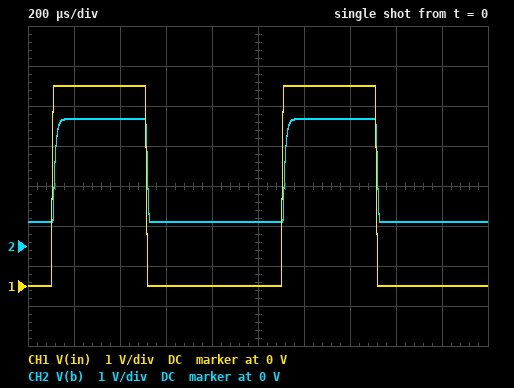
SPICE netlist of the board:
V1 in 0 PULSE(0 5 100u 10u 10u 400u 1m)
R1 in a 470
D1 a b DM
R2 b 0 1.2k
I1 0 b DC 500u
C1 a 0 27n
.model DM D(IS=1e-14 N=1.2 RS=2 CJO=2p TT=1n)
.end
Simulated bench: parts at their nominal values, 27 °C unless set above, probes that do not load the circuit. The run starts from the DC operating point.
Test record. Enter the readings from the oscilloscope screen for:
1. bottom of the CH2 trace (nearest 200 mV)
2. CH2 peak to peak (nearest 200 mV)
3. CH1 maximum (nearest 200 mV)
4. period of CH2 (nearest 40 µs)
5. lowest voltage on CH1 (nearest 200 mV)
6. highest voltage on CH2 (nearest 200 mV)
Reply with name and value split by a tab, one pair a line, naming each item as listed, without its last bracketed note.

bottom of the CH2 trace	600 mV
CH2 peak to peak	2.6 V
CH1 maximum	5.0 V
period of CH2	1.00 ms
lowest voltage on CH1	0 V
highest voltage on CH2	3.2 V
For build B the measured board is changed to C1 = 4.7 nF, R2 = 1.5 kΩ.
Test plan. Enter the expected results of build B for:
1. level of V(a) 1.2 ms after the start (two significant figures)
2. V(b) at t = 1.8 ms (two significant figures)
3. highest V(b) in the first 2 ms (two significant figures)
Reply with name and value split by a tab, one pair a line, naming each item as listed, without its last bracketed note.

level of V(a) 1.2 ms after the start	4.2 V
V(b) at t = 1.8 ms	750 mV
highest V(b) in the first 2 ms	3.4 V
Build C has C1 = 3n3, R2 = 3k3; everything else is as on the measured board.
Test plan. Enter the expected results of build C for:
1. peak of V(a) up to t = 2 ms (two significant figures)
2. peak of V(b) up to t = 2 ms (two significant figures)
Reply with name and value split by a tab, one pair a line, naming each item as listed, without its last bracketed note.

peak of V(a) up to t = 2 ms	4.7 V
peak of V(b) up to t = 2 ms	3.9 V
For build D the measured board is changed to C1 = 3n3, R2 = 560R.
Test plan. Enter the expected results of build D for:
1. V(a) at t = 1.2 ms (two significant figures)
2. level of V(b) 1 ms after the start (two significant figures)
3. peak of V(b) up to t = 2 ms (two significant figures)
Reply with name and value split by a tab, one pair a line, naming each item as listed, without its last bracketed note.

V(a) at t = 1.2 ms	3.2 V
level of V(b) 1 ms after the start	280 mV
peak of V(b) up to t = 2 ms	2.4 V
